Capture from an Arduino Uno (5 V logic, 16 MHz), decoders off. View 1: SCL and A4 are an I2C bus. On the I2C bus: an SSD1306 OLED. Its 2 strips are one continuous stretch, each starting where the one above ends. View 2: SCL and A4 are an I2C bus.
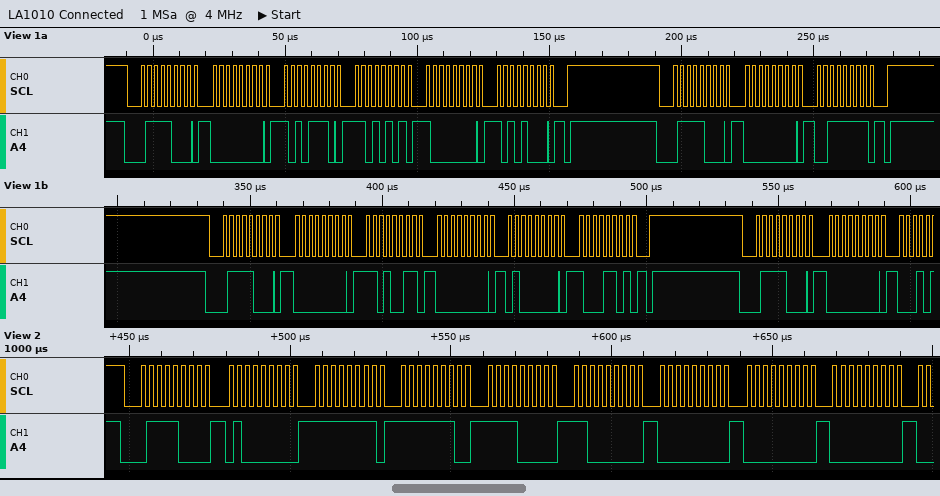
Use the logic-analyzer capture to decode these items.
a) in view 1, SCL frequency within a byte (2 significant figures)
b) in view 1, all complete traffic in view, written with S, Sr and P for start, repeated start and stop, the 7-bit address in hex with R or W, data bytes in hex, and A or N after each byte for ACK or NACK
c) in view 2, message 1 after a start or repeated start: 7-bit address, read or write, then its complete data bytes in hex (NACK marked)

400 kHz
S 3CW A 00 A AE A D5 A 80 A A8 A P S 3CW A 00 A 3F A P S 3CW A 00 A D3 A 00 A 40 A 8D A P S 3CW A 00 A
0x3C write: 40 FF FE F0 C0 00 00 00
